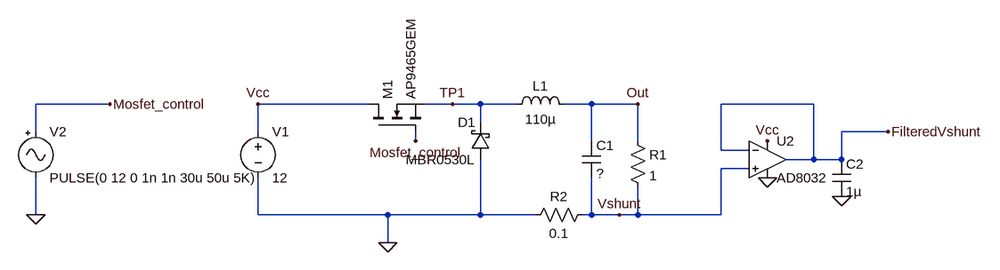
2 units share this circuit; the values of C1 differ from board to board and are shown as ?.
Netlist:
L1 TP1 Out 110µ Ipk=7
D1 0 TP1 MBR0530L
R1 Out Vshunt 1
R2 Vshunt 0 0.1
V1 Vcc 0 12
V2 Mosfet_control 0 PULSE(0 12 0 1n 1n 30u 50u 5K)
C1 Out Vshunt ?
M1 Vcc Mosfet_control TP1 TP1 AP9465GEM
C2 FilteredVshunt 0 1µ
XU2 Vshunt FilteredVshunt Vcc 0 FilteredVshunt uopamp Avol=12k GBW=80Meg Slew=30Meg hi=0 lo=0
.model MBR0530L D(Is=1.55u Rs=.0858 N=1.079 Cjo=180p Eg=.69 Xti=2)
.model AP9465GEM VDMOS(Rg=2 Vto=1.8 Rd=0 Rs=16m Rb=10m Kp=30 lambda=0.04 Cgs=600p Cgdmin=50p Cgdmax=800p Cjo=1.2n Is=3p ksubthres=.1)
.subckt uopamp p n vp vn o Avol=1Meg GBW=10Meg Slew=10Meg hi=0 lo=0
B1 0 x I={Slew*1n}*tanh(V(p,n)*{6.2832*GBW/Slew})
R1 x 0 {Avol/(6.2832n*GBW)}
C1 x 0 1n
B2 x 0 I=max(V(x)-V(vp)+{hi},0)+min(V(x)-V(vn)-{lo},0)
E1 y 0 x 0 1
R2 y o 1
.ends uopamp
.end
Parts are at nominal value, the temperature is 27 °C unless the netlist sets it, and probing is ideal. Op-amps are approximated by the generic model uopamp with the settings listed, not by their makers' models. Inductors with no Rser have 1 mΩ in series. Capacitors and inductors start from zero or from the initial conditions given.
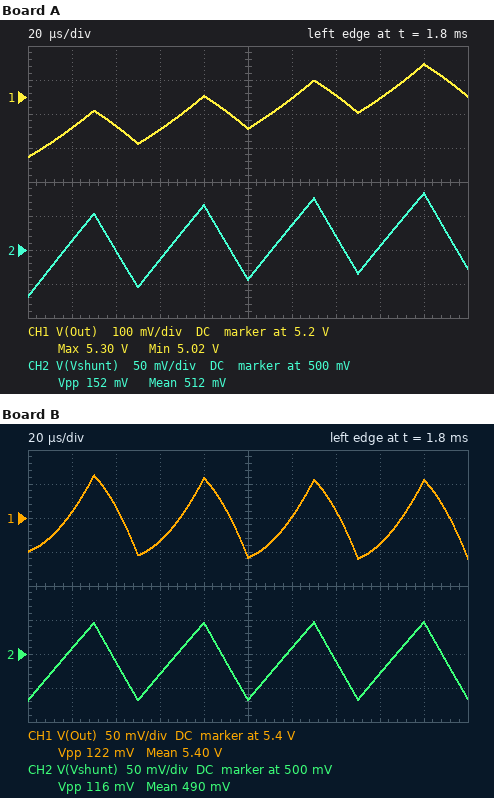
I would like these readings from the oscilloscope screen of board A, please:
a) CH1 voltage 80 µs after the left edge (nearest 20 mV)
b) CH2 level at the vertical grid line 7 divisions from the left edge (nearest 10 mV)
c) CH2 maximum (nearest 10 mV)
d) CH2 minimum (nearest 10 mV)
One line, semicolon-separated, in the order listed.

5.20 V; 520 mV; 580 mV; 430 mV
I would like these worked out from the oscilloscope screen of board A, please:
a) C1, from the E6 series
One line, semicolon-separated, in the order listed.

680 µF
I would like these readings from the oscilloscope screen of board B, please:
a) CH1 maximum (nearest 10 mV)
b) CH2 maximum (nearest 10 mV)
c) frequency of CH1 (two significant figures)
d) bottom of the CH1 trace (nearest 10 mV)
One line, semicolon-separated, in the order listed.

5.46 V; 550 mV; 20 kHz; 5.34 V
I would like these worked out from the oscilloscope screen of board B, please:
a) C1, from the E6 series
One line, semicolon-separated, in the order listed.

220 µF
